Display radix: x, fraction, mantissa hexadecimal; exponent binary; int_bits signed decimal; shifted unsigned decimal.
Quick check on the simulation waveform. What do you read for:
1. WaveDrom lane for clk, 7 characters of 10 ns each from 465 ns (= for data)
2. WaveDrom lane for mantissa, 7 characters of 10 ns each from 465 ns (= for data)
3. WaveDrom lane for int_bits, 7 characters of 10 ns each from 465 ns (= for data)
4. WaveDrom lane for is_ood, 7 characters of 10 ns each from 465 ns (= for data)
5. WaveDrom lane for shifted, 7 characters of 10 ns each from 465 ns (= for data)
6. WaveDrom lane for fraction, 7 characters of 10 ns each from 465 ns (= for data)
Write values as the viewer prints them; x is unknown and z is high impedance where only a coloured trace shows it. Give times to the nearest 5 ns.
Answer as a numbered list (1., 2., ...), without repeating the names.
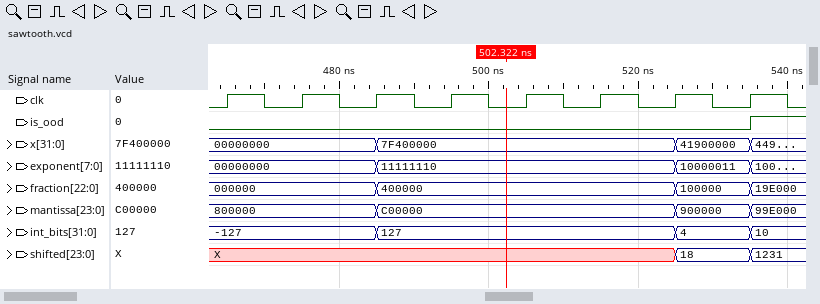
1. {name: 'clk', wave: 'p......'}
2. {name: 'mantissa', wave: '=.=...=', data: '800000 C00000 900000'}
3. {name: 'int_bits', wave: '=.=...=', data: '-127 127 4'}
4. {name: 'is_ood', wave: '0......'}
5. {name: 'shifted', wave: 'x.....=', data: '18'}
6. {name: 'fraction', wave: '=.=...=', data: '000000 400000 100000'}
